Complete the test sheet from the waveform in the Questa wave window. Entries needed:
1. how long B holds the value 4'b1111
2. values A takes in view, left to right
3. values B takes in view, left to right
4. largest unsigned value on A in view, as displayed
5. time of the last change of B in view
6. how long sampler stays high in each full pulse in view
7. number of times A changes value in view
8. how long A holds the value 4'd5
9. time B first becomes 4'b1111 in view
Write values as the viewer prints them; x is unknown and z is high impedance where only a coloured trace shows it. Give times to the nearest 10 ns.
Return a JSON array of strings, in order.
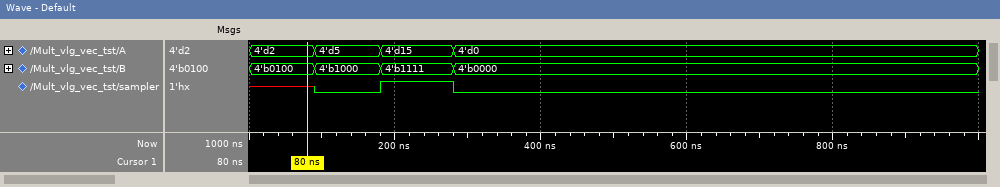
["100 ns", "4'd2, 4'd5, 4'd15, 4'd0", "4'b0100, 4'b1000, 4'b1111, 4'b0000", "4'd15", "280 ns", "100 ns", "3", "90 ns", "180 ns"]
